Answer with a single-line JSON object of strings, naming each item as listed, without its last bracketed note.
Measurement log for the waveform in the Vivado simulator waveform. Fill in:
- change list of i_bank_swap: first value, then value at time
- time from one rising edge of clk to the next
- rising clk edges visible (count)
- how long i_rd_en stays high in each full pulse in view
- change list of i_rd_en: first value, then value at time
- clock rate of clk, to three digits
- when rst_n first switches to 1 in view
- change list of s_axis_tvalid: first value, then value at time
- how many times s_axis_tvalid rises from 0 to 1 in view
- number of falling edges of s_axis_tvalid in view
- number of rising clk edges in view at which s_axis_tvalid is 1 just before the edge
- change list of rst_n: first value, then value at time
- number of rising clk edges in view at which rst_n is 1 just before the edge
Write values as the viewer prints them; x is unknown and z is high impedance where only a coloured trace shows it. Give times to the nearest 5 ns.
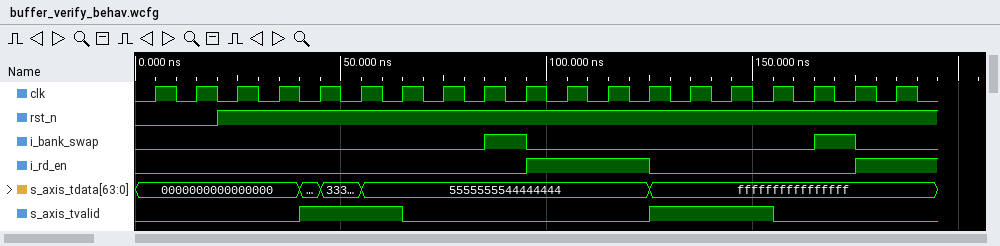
{"change list of i_bank_swap: first value, then value at time": "0, 1 at 85 ns, 0 at 95 ns, 1 at 165 ns, 0 at 175 ns", "time from one rising edge of clk to the next": "10 ns", "rising clk edges visible": "19", "how long i_rd_en stays high in each full pulse in view": "30 ns", "change list of i_rd_en: first value, then value at time": "0, 1 at 95 ns, 0 at 125 ns, 1 at 175 ns", "clock rate of clk, to three digits": "100 MHz", "when rst_n first switches to 1 in view": "20 ns", "change list of s_axis_tvalid: first value, then value at time": "0, 1 at 40 ns, 0 at 65 ns, 1 at 125 ns, 0 at 155 ns", "how many times s_axis_tvalid rises from 0 to 1 in view": "2", "number of falling edges of s_axis_tvalid in view": "2", "number of rising clk edges in view at which s_axis_tvalid is 1 just before the edge": "6", "change list of rst_n: first value, then value at time": "0, 1 at 20 ns", "number of rising clk edges in view at which rst_n is 1 just before the edge": "17"}
